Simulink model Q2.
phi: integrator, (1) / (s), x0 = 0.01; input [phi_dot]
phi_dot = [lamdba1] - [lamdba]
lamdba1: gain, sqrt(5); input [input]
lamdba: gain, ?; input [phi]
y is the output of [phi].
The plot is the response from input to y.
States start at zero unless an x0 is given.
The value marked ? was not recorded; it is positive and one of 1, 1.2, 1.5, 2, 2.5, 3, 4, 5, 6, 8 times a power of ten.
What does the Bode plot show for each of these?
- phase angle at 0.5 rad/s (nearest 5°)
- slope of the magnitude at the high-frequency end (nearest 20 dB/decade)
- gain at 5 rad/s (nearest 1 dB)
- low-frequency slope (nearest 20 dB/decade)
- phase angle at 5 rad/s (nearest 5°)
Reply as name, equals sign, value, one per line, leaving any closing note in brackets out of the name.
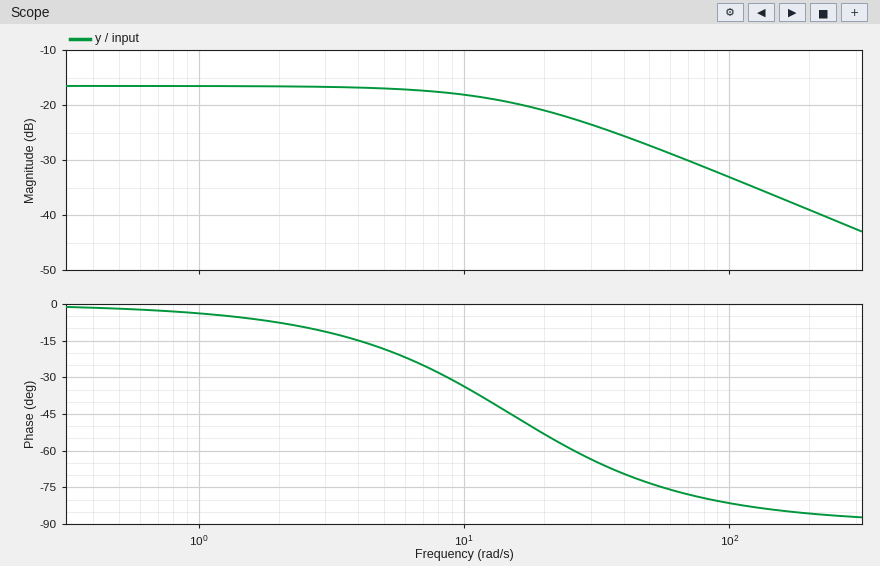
phase angle at 0.5 rad/s = 0°
slope of the magnitude at the high-frequency end = -20 dB/decade
gain at 5 rad/s = -17 dB
low-frequency slope = 0 dB/decade
phase angle at 5 rad/s = -20°
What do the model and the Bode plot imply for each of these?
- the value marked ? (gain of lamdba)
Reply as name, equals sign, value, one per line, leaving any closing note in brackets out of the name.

the value marked ? = 15
